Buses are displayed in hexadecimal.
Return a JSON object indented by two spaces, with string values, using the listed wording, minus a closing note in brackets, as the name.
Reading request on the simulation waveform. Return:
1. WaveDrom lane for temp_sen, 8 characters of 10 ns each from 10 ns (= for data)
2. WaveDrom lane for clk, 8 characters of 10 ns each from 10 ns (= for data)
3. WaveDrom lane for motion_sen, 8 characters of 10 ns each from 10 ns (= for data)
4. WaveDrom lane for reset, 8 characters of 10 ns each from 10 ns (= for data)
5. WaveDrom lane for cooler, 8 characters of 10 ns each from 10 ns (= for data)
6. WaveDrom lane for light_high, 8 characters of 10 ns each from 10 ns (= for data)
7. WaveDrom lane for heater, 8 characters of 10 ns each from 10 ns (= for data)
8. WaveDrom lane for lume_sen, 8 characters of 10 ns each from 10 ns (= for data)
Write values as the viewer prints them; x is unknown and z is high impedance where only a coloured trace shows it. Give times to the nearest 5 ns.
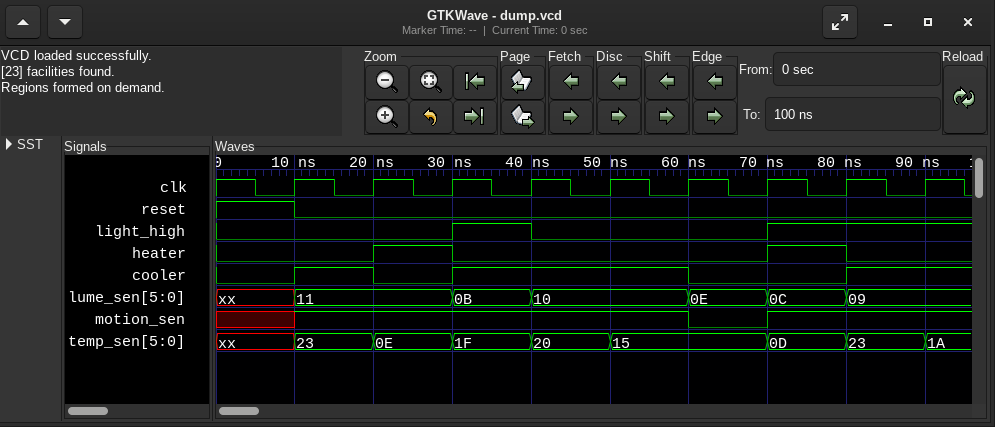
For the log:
{
  "WaveDrom lane for temp_sen, 8 characters of 10 ns each from 10 ns": "{name: 'temp_sen', wave: '=====.==', data: '23 0E 1F 20 15 0D 23'}",
  "WaveDrom lane for clk, 8 characters of 10 ns each from 10 ns": "{name: 'clk', wave: 'p.......'}",
  "WaveDrom lane for motion_sen, 8 characters of 10 ns each from 10 ns": "{name: 'motion_sen', wave: '1....01.'}",
  "WaveDrom lane for reset, 8 characters of 10 ns each from 10 ns": "{name: 'reset', wave: '0.......'}",
  "WaveDrom lane for cooler, 8 characters of 10 ns each from 10 ns": "{name: 'cooler', wave: '101..0.1'}",
  "WaveDrom lane for light_high, 8 characters of 10 ns each from 10 ns": "{name: 'light_high', wave: '0.10..1.'}",
  "WaveDrom lane for heater, 8 characters of 10 ns each from 10 ns": "{name: 'heater', wave: '010...10'}",
  "WaveDrom lane for lume_sen, 8 characters of 10 ns each from 10 ns": "{name: 'lume_sen', wave: '=.==.===', data: '11 0B 10 0E 0C 09'}"
}
